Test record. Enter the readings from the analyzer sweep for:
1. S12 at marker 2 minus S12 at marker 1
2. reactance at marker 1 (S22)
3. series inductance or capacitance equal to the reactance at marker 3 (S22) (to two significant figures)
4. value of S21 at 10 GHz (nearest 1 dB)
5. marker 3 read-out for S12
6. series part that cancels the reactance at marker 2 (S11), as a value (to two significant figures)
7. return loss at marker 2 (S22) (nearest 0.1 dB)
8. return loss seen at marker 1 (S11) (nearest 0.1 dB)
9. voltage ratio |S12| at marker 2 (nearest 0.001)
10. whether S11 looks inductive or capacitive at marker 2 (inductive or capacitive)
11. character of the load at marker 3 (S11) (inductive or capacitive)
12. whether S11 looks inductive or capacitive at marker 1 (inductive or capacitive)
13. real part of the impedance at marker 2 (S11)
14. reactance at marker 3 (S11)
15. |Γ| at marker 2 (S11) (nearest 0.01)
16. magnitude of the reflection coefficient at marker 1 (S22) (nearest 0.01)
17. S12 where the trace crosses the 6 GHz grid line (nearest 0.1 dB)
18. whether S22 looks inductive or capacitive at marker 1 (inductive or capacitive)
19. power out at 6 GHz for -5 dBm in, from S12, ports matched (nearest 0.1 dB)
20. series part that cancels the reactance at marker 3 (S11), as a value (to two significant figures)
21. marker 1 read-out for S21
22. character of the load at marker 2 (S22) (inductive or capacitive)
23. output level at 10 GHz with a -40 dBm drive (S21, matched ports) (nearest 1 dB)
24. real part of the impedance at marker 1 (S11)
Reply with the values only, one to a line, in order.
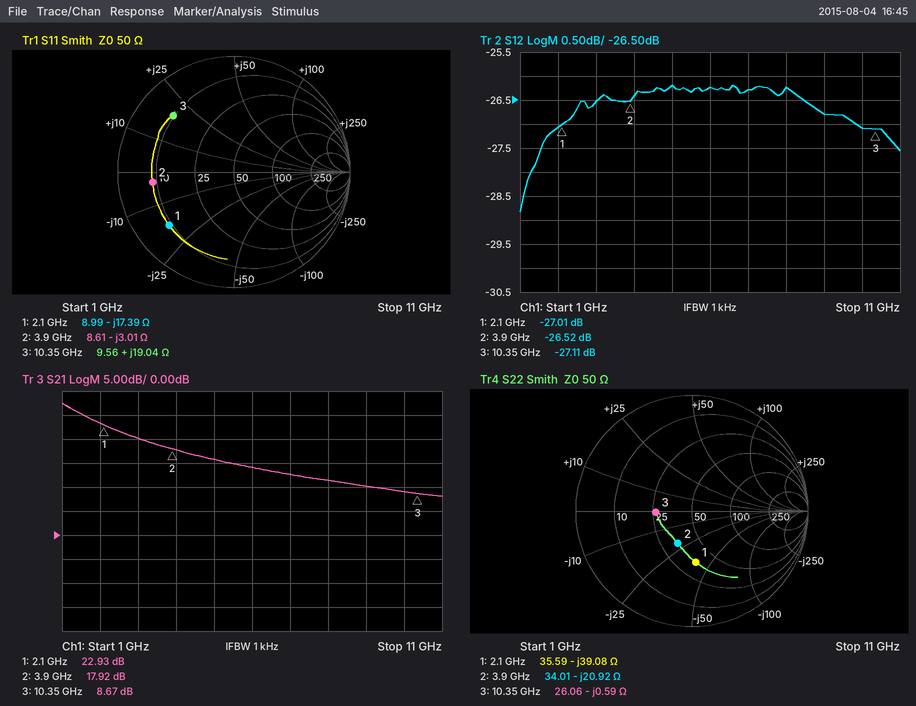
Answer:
0.49 dB
-39.08 Ω
26 pF
9 dB
-27.11 dB
120 pH
10.3 dB
2.8 dB
0.047
capacitive
inductive
capacitive
8.61 Ω
+19.04 Ω
0.71
0.44
-26.2 dB
capacitive
-31.2 dBm
810 fF
22.93 dB
capacitive
-31 dBm
8.99 Ω
